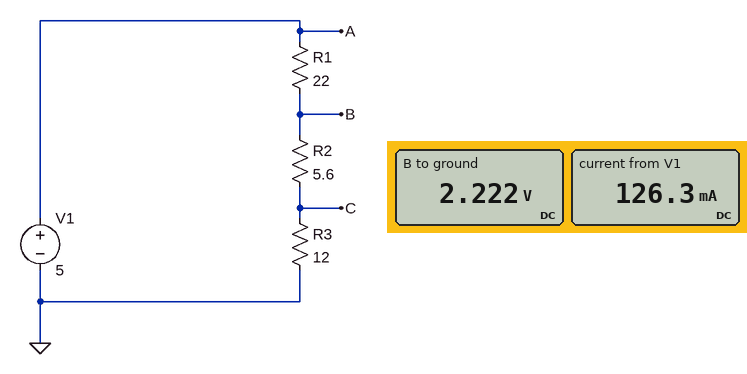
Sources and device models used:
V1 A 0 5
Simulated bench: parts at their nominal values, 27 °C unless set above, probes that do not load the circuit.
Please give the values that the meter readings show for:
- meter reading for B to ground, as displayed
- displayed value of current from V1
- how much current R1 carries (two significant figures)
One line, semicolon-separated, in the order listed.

2.222 V; 126.3 mA; 130 mA
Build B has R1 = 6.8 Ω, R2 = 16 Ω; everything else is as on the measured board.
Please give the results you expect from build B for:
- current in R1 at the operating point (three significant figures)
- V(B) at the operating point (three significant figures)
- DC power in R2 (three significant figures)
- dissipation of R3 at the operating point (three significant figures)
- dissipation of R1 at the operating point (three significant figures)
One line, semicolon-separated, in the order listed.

144 mA; 4.02 V; 330 mW; 248 mW; 140 mW
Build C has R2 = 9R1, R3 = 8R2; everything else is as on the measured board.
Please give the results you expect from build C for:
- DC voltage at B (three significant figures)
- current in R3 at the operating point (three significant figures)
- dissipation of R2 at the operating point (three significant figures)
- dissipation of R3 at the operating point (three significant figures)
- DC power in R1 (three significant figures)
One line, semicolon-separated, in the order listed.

2.20 V; 127 mA; 147 mW; 133 mW; 356 mW
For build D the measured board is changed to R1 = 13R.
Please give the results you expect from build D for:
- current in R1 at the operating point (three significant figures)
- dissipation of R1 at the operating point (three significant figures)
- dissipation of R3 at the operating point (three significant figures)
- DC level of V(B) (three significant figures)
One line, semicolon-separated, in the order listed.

163 mA; 347 mW; 320 mW; 2.88 V
